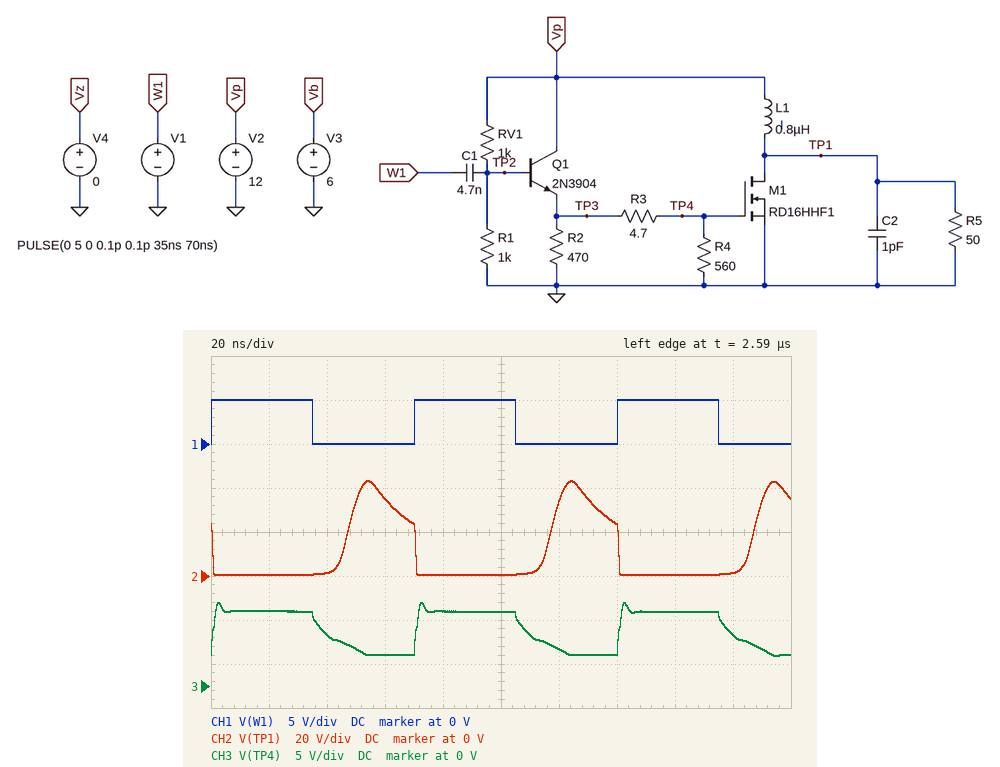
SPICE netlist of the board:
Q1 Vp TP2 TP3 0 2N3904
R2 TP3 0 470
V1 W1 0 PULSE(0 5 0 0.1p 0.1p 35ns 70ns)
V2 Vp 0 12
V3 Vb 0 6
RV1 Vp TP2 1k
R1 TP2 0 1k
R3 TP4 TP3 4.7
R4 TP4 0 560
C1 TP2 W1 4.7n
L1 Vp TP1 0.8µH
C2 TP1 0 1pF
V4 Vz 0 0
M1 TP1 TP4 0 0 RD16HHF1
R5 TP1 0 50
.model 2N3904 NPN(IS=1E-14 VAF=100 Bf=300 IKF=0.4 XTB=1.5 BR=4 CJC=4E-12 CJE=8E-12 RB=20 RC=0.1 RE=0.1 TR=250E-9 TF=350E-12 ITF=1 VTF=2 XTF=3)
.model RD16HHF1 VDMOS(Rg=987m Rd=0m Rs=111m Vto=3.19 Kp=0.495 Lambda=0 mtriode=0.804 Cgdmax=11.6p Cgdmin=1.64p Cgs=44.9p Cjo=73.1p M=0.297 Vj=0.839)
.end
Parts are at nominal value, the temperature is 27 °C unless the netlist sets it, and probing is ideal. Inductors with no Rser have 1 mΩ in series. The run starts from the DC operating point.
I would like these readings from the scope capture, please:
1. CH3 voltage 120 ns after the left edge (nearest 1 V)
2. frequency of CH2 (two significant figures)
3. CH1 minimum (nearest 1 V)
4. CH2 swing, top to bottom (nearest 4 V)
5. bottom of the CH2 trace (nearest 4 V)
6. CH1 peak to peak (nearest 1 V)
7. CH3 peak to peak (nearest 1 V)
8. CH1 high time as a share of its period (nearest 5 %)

4 V
14 MHz
0 V
44 V
0 V
5 V
6 V
50 %
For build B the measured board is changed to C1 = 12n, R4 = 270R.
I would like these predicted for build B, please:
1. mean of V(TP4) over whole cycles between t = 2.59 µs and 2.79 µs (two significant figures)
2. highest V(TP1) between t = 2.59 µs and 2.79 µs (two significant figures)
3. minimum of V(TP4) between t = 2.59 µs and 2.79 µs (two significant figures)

6.9 V
42 V
4.2 V
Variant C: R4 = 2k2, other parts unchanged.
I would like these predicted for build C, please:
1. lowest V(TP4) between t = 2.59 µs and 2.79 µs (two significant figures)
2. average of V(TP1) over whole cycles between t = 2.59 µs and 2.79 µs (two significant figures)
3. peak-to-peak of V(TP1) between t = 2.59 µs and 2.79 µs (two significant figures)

3.5 V
12 V
47 V
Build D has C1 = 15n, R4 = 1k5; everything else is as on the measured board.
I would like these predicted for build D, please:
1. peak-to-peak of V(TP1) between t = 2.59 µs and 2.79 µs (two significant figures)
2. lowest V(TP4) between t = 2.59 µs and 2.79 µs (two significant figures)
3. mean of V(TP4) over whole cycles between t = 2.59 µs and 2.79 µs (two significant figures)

49 V
4.4 V
7.5 V
